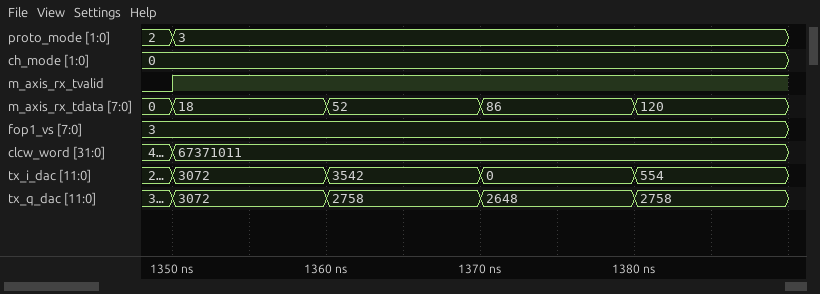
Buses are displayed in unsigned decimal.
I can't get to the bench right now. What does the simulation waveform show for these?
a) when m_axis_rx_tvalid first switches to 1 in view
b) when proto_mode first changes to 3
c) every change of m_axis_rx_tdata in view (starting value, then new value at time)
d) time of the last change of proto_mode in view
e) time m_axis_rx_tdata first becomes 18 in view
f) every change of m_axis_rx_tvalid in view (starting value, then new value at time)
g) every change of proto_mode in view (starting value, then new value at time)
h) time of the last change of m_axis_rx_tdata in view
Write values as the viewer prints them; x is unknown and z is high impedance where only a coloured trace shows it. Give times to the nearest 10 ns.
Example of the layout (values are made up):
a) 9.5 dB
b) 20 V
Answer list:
a) 1350 ns
b) 1350 ns
c) 0, 18 at 1350 ns, 52 at 1360 ns, 86 at 1370 ns, 120 at 1380 ns
d) 1350 ns
e) 1350 ns
f) 0, 1 at 1350 ns
g) 2, 3 at 1350 ns
h) 1380 ns
